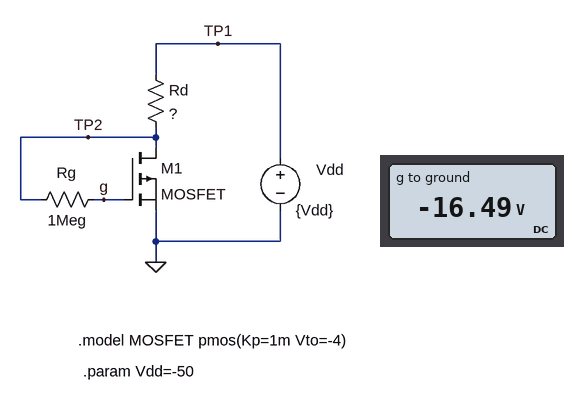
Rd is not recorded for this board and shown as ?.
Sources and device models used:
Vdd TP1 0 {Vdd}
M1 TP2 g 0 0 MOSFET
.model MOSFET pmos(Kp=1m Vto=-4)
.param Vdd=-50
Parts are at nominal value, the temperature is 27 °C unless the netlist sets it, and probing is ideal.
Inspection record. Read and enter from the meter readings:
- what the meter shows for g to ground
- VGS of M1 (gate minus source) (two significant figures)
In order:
-16.49 V
-16 V
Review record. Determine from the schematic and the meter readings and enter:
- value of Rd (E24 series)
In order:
430 Ω
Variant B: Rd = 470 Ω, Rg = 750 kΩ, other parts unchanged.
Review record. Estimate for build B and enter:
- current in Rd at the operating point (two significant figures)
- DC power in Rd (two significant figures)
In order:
72 mA
2.5 W
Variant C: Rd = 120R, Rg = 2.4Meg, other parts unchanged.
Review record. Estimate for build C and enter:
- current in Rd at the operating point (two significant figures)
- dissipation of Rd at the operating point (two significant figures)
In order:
210 mA
5.4 W
